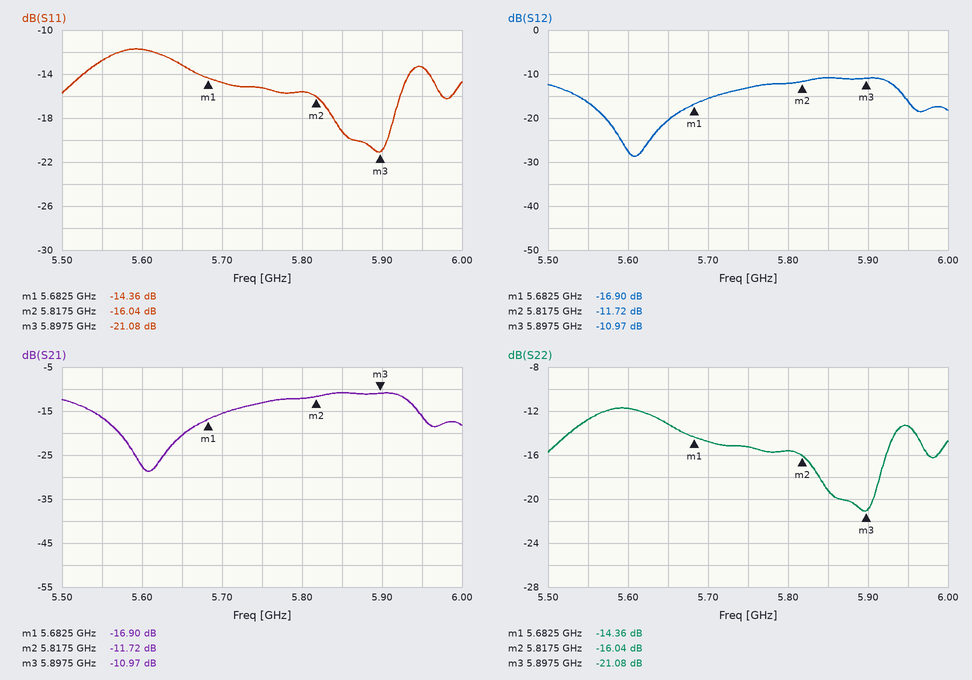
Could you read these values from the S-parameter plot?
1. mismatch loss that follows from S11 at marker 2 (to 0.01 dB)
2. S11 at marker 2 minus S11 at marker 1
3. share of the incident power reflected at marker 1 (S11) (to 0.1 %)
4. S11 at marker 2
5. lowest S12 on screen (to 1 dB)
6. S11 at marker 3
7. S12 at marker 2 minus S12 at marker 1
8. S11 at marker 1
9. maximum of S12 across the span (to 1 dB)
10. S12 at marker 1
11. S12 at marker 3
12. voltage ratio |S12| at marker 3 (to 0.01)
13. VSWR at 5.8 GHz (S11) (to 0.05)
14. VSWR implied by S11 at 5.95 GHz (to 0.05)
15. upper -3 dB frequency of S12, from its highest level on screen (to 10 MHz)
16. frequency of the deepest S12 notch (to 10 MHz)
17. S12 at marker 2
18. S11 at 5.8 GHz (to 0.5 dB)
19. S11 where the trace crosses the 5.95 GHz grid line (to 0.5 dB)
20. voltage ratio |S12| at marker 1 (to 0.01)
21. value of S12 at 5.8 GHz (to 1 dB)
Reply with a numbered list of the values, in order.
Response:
1. 0.11 dB
2. -1.68 dB
3. 3.7 %
4. -16.04 dB
5. -29 dB
6. -21.08 dB
7. 5.18 dB
8. -14.36 dB
9. -11 dB
10. -16.90 dB
11. -10.97 dB
12. 0.28
13. 1.40
14. 1.55
15. 5.94 GHz
16. 5.61 GHz
17. -11.72 dB
18. -15.5 dB
19. -13.5 dB
20. 0.14
21. -12 dB
